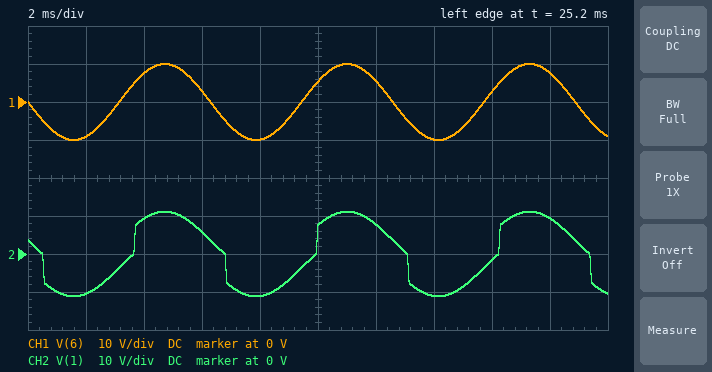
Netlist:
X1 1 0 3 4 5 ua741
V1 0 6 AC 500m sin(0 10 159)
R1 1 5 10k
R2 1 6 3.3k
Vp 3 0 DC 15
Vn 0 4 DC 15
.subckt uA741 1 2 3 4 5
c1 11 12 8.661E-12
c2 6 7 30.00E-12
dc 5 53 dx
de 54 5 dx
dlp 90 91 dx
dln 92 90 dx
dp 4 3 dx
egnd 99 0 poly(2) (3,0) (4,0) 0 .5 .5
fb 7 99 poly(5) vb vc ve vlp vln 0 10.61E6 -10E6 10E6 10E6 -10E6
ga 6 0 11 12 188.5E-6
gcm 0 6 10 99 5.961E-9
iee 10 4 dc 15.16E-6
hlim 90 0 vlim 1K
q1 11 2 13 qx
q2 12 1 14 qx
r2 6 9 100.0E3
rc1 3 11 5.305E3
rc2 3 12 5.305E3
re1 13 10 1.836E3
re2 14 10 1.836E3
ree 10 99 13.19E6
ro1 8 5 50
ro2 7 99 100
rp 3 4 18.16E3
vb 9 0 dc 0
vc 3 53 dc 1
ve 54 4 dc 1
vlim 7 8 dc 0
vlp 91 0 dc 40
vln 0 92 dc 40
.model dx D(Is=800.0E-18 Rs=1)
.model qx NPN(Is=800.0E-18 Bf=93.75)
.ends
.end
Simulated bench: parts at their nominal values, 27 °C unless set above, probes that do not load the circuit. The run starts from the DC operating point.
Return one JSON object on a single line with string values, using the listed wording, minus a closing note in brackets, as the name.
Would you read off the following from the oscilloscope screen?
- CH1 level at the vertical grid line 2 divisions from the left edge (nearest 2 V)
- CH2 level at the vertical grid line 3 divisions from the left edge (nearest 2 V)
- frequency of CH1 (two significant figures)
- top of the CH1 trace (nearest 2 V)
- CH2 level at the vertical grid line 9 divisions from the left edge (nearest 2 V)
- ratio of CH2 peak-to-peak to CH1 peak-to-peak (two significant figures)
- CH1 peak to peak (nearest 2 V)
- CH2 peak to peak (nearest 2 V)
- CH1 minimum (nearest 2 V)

{"CH1 level at the vertical grid line 2 divisions from the left edge": "8 V", "CH2 level at the vertical grid line 3 divisions from the left edge": "6 V", "frequency of CH1": "160 Hz", "top of the CH1 trace": "10 V", "CH2 level at the vertical grid line 9 divisions from the left edge": "10 V", "ratio of CH2 peak-to-peak to CH1 peak-to-peak": "1.1", "CH1 peak to peak": "20 V", "CH2 peak to peak": "22 V", "CH1 minimum": "-10 V"}
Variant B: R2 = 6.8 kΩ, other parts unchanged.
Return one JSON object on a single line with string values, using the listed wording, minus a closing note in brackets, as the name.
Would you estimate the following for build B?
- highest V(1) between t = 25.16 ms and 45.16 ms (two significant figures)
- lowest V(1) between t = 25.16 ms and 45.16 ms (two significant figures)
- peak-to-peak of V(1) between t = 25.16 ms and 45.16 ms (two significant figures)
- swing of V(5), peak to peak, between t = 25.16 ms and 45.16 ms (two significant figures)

{"highest V(1) between t = 25.16 ms and 45.16 ms": "12 V", "lowest V(1) between t = 25.16 ms and 45.16 ms": "-12 V", "peak-to-peak of V(1) between t = 25.16 ms and 45.16 ms": "24 V", "swing of V(5), peak to peak, between t = 25.16 ms and 45.16 ms": "29 V"}
